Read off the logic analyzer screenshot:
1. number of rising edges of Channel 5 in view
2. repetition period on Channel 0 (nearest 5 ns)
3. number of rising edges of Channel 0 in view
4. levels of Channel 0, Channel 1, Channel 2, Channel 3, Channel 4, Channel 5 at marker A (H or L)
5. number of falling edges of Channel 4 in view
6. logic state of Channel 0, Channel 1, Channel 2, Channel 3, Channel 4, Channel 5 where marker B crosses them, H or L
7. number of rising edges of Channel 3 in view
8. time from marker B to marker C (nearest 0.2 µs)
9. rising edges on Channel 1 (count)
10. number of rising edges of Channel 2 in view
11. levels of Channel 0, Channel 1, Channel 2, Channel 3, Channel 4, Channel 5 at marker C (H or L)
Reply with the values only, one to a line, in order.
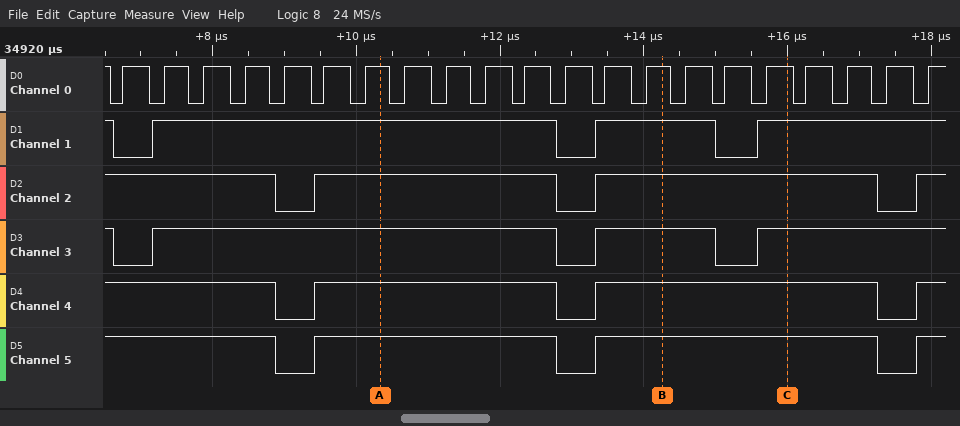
3
560 ns
21
Channel 0=H, Channel 1=H, Channel 2=H, Channel 3=H, Channel 4=H, Channel 5=H
3
Channel 0=H, Channel 1=H, Channel 2=H, Channel 3=H, Channel 4=H, Channel 5=H
3
1.8 µs
3
3
Channel 0=H, Channel 1=H, Channel 2=H, Channel 3=H, Channel 4=H, Channel 5=H
